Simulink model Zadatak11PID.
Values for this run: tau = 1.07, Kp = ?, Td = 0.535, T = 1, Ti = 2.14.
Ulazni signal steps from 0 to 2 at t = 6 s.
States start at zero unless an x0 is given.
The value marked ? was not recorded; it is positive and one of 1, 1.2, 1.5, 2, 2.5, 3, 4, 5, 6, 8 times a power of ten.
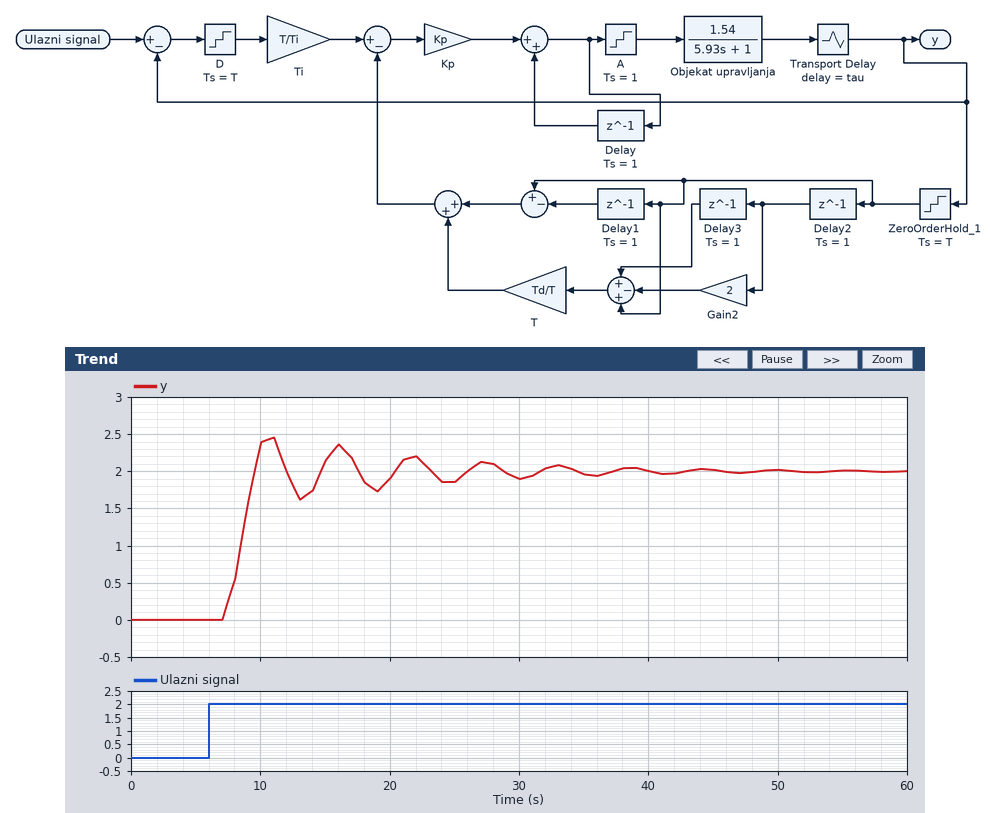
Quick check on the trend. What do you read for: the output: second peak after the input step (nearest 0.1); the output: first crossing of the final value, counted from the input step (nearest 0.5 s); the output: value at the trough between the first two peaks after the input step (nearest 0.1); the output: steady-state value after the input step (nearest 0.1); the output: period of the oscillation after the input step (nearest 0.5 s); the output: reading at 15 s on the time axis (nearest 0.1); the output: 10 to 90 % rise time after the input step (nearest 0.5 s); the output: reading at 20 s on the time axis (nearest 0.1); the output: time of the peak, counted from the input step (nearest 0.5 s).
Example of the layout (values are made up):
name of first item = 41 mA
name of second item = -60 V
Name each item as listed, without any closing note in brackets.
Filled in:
the output: second peak after the input step = 2.4
the output: first crossing of the final value, counted from the input step = 3.5 s
the output: value at the trough between the first two peaks after the input step = 1.6
the output: steady-state value after the input step = 2.0
the output: period of the oscillation after the input step = 5.0 s
the output: reading at 15 s on the time axis = 2.1
the output: 10 to 90 % rise time after the input step = 2.0 s
the output: reading at 20 s on the time axis = 1.9
the output: time of the peak, counted from the input step = 5.0 s
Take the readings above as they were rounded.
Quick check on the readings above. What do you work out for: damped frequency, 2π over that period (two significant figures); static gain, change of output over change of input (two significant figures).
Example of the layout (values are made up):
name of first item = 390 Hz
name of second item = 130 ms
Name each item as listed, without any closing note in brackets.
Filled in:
damped frequency, 2π over that period = 1.3 rad/s
static gain, change of output over change of input = 1.0
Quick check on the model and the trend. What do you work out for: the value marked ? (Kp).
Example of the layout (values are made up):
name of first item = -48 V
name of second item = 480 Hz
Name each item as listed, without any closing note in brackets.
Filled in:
the value marked ? = 2.5
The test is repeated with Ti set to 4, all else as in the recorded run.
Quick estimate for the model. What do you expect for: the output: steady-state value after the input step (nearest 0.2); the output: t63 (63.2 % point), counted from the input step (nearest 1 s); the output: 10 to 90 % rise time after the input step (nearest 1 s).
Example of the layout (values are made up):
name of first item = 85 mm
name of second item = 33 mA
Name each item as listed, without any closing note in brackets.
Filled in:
the output: steady-state value after the input step = 2.0
the output: t63 (63.2 % point), counted from the input step = 4 s
the output: 10 to 90 % rise time after the input step = 7 s
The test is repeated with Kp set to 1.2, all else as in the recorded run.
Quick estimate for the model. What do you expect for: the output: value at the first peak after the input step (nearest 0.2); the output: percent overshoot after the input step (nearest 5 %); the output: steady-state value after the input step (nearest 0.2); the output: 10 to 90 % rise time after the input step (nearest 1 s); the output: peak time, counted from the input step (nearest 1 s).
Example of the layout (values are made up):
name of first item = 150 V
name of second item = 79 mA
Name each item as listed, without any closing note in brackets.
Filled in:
the output: value at the first peak after the input step = 2.4
the output: percent overshoot after the input step = 15 %
the output: steady-state value after the input step = 2.0
the output: 10 to 90 % rise time after the input step = 3 s
the output: peak time, counted from the input step = 8 s
